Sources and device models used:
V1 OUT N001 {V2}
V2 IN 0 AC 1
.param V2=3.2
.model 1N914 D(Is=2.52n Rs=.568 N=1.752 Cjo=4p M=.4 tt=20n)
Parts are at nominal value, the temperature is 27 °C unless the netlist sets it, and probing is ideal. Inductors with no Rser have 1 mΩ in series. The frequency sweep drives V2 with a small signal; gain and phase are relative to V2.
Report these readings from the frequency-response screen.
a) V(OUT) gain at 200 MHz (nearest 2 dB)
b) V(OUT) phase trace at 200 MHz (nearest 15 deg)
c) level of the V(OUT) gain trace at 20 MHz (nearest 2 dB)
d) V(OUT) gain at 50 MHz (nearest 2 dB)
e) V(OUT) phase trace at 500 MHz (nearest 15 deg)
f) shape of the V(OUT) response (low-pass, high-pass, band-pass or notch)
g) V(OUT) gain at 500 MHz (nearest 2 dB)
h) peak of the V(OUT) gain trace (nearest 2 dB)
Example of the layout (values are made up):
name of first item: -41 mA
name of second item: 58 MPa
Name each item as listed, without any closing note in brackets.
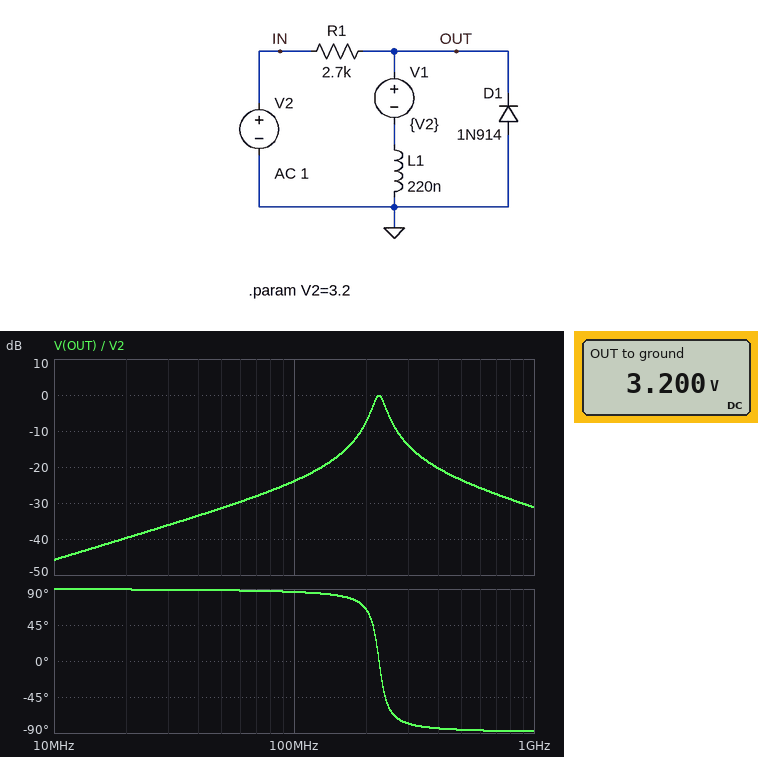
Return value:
V(OUT) gain at 200 MHz: -8 dB
V(OUT) phase trace at 200 MHz: 60 deg
level of the V(OUT) gain trace at 20 MHz: -40 dB
V(OUT) gain at 50 MHz: -32 dB
V(OUT) phase trace at 500 MHz: -90 deg
shape of the V(OUT) response: band-pass
V(OUT) gain at 500 MHz: -24 dB
peak of the V(OUT) gain trace: 0 dB
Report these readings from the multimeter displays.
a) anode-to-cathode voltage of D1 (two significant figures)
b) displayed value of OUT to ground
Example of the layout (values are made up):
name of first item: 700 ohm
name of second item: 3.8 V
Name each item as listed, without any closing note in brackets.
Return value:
anode-to-cathode voltage of D1: -3.2 V
displayed value of OUT to ground: 3.200 V
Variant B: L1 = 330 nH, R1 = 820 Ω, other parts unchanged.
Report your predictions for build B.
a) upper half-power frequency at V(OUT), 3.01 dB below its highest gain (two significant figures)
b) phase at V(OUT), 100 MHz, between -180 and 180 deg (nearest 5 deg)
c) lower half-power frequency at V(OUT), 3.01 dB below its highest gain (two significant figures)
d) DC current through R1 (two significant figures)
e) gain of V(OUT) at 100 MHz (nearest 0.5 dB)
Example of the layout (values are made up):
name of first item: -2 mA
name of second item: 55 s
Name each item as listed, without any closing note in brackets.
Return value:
upper half-power frequency at V(OUT), 3.01 dB below its highest gain: 230 MHz
phase at V(OUT), 100 MHz, between -180 and 180 deg: 70 deg
lower half-power frequency at V(OUT), 3.01 dB below its highest gain: 150 MHz
DC current through R1: 3.9 mA
gain of V(OUT) at 100 MHz: -9.5 dB
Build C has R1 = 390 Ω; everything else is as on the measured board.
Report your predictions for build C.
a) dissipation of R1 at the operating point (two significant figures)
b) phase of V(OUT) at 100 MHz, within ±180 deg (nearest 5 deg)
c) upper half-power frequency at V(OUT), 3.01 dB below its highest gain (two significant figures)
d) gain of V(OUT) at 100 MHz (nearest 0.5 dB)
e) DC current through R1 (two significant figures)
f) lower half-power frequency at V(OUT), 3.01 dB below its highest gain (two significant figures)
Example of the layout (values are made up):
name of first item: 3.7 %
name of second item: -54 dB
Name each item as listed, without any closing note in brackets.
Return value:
dissipation of R1 at the operating point: 26 mW
phase of V(OUT) at 100 MHz, within ±180 deg: 65 deg
upper half-power frequency at V(OUT), 3.01 dB below its highest gain: 330 MHz
gain of V(OUT) at 100 MHz: -8.0 dB
DC current through R1: 8.2 mA
lower half-power frequency at V(OUT), 3.01 dB below its highest gain: 150 MHz
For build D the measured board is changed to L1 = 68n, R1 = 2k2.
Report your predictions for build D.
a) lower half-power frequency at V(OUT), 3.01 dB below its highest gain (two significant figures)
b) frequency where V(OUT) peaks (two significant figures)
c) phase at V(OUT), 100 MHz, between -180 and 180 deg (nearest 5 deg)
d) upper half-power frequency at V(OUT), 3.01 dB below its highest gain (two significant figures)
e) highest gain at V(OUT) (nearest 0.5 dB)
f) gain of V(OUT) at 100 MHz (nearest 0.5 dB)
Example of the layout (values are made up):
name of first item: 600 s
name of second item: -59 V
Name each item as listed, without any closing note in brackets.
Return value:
lower half-power frequency at V(OUT), 3.01 dB below its highest gain: 390 MHz
frequency where V(OUT) peaks: 410 MHz
phase at V(OUT), 100 MHz, between -180 and 180 deg: 90 deg
upper half-power frequency at V(OUT), 3.01 dB below its highest gain: 420 MHz
highest gain at V(OUT): -0.5 dB
gain of V(OUT) at 100 MHz: -33.5 dB
